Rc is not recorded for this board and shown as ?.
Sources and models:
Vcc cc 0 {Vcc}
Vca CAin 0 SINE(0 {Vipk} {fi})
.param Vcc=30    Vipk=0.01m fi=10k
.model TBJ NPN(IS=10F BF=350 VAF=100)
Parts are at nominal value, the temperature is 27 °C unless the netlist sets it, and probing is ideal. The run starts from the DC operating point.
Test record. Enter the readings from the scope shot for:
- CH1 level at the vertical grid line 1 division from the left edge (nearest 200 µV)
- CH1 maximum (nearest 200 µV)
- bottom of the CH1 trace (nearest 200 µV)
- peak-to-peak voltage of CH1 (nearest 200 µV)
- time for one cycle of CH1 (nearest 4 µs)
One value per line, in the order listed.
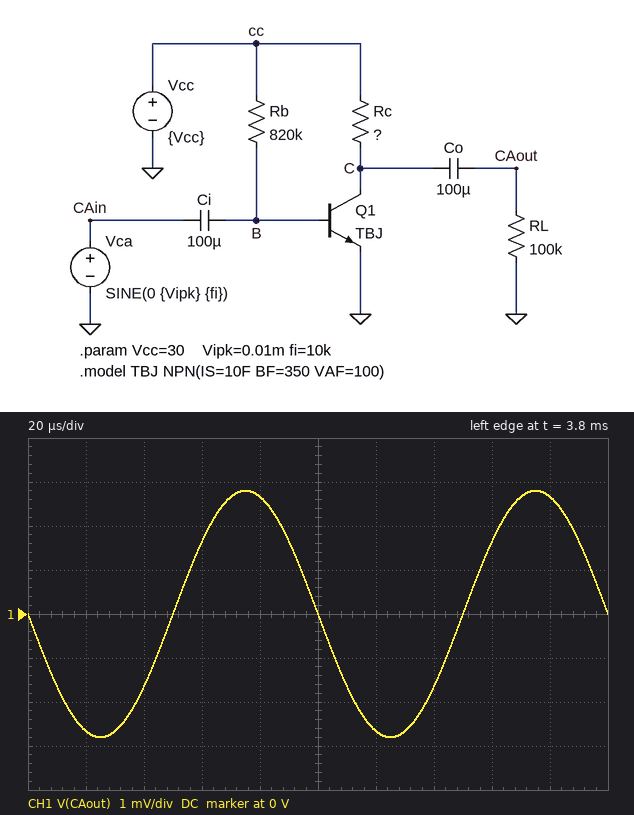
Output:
-2.6 mV
2.8 mV
-2.8 mV
5.6 mV
100 µs
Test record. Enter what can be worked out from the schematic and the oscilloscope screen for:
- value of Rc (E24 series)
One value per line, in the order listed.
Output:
510 Ω
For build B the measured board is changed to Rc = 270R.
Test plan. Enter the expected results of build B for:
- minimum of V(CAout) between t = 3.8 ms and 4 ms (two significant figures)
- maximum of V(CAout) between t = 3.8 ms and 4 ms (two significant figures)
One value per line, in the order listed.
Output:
-1.6 mV
1.6 mV
